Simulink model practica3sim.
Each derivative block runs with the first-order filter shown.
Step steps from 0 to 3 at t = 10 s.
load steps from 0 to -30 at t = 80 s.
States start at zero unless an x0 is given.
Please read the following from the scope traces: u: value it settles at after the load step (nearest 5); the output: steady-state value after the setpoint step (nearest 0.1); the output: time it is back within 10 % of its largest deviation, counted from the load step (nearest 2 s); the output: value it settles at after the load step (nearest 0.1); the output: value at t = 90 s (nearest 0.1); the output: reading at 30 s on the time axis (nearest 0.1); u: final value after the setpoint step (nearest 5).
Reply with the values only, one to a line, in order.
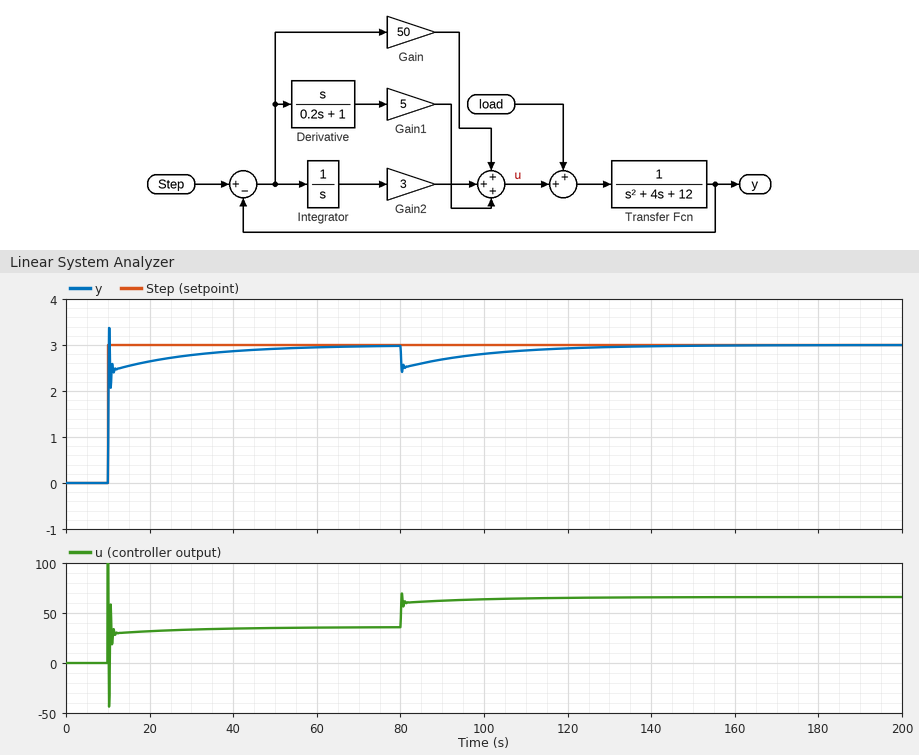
65
3.0
46 s
3.0
2.7
2.8
35
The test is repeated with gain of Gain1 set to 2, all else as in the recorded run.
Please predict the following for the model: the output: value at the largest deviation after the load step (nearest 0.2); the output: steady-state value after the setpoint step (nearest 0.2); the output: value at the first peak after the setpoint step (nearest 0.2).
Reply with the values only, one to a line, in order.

2.4
3.0
3.4
